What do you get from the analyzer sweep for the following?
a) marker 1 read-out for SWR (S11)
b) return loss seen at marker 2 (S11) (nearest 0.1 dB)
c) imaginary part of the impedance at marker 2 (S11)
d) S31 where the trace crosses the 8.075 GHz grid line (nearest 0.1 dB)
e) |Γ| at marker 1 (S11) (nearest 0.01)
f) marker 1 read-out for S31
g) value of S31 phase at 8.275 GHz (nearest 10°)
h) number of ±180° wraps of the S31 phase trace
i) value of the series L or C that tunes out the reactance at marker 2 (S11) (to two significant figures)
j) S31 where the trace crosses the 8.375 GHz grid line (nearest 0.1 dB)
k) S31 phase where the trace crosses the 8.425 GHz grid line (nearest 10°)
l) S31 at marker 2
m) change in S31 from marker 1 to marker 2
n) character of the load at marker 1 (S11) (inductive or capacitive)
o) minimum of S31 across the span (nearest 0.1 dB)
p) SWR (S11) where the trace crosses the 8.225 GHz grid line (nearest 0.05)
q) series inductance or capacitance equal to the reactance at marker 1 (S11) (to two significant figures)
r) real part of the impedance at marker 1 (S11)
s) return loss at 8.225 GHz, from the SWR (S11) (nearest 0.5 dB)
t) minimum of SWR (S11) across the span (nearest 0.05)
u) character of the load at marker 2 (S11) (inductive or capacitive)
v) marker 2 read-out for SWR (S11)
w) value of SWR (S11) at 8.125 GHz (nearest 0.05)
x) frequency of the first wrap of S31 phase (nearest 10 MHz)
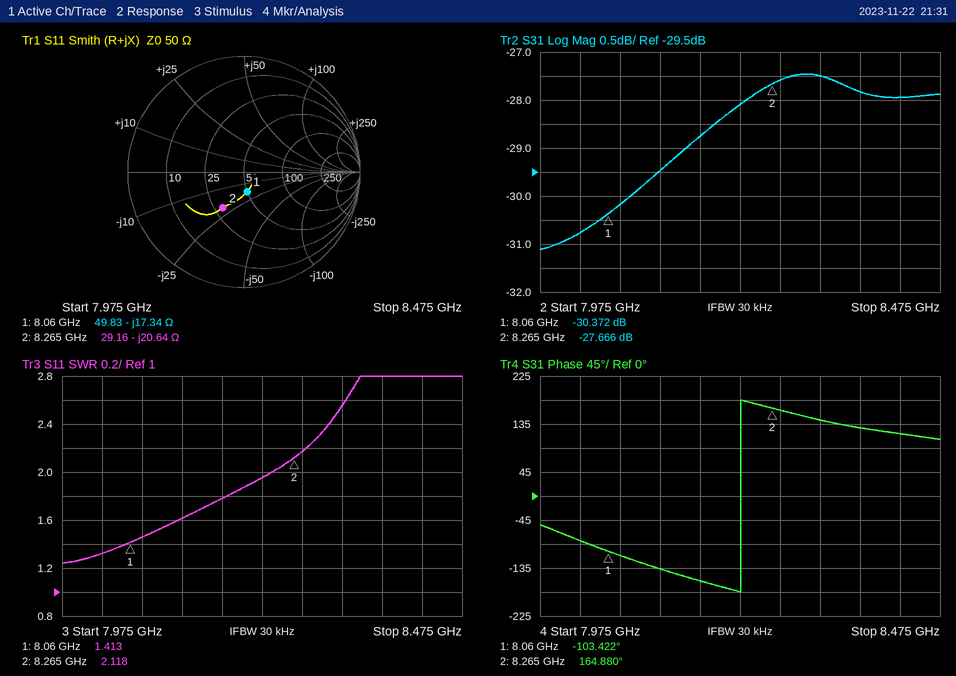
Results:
1.413
8.9 dB
-20.64 Ω
-30.2 dB
0.17
-30.372 dB
160°
1
400 pH
-27.8 dB
120°
-27.666 dB
2.706 dB
capacitive
-31.1 dB
1.95
1.1 pF
49.83 Ω
10.0 dB
1.25
capacitive
2.118
1.60
8.23 GHz
